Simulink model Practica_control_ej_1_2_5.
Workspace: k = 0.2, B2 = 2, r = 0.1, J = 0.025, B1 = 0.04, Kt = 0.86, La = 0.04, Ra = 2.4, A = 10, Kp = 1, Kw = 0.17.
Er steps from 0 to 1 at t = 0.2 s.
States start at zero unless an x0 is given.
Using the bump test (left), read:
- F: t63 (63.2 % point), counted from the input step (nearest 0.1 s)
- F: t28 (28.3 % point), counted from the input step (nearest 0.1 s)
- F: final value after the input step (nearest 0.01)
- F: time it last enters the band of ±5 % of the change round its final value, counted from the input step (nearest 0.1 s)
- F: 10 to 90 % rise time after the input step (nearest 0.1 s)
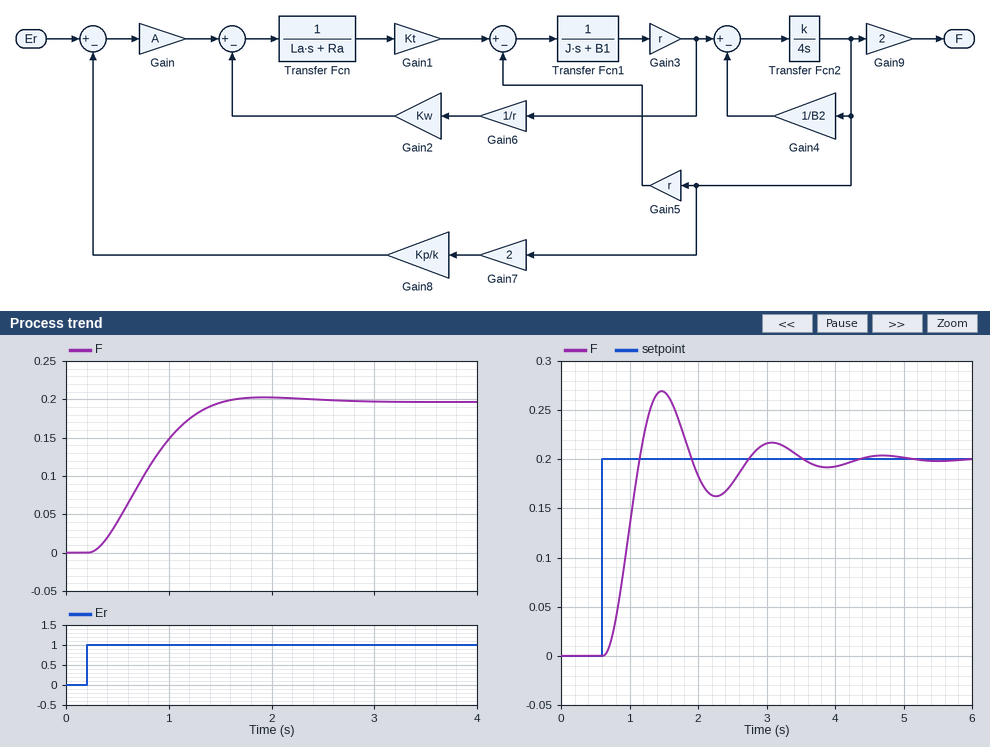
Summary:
0.7 s
0.4 s
0.20
1.1 s
0.8 s
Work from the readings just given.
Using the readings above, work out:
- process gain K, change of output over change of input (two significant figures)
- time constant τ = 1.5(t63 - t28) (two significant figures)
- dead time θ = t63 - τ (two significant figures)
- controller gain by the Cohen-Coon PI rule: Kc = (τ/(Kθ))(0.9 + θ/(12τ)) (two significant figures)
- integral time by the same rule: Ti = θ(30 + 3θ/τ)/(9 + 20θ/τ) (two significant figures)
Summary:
0.20
0.45 s
0.25 s
8.5
0.39 s
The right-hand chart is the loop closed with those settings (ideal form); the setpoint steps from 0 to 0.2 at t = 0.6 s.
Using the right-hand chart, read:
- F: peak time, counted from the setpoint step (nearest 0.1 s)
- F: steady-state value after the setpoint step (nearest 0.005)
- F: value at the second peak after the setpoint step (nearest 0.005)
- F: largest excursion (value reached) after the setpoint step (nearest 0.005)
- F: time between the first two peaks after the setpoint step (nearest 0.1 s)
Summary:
0.9 s
0.200
0.215
0.270
1.6 s
